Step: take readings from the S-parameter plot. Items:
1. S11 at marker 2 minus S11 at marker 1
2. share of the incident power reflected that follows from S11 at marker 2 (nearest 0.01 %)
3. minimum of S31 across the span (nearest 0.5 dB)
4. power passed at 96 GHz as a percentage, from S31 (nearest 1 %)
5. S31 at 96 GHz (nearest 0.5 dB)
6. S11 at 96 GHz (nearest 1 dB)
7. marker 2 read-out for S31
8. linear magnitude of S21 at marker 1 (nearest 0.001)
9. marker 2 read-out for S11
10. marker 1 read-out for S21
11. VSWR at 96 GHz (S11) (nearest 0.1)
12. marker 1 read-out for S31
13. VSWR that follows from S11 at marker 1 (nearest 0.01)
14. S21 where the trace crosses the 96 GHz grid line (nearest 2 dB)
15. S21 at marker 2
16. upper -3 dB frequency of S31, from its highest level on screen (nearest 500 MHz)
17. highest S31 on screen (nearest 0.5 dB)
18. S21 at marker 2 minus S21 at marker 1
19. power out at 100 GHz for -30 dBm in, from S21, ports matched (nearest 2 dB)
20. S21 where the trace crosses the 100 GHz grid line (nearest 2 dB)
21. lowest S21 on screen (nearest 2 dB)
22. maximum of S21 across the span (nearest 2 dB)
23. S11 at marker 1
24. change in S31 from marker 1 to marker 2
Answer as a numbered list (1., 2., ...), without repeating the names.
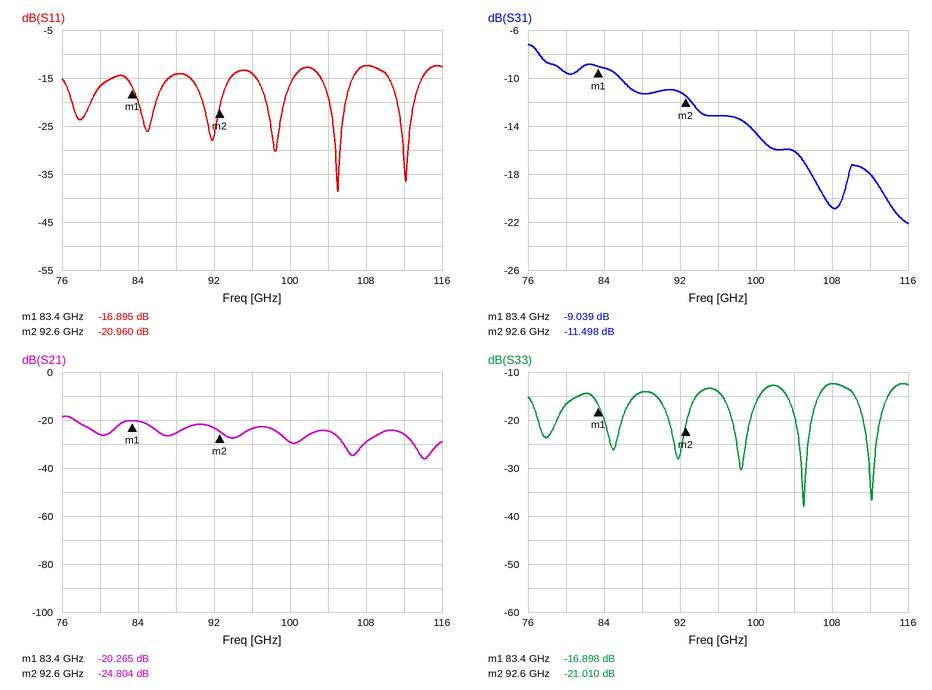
1. -4.065 dB
2. 0.80 %
3. -22.0 dB
4. 5 %
5. -13.0 dB
6. -14 dB
7. -11.498 dB
8. 0.097
9. -20.960 dB
10. -20.265 dB
11. 1.5
12. -9.039 dB
13. 1.33
14. -24 dB
15. -24.804 dB
16. 86.0 GHz
17. -7.0 dB
18. -4.539 dB
19. -60 dBm
20. -30 dB
21. -36 dB
22. -18 dB
23. -16.895 dB
24. -2.459 dB
